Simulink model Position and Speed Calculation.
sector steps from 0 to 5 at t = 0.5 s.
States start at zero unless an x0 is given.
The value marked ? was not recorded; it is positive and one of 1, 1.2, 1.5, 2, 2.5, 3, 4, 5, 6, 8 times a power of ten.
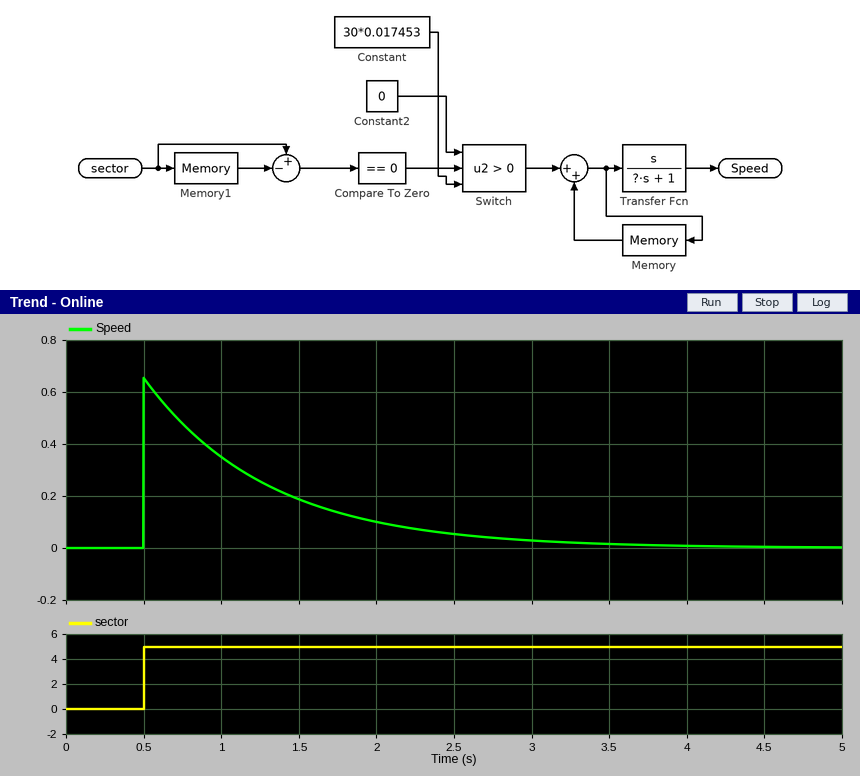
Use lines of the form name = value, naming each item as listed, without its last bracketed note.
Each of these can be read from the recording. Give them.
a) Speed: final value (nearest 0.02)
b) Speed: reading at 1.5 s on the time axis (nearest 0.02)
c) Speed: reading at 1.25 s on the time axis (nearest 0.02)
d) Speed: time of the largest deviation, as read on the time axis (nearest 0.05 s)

Speed: final value = 0.00
Speed: reading at 1.5 s on the time axis = 0.18
Speed: reading at 1.25 s on the time axis = 0.26
Speed: time of the largest deviation, as read on the time axis = 0.50 s
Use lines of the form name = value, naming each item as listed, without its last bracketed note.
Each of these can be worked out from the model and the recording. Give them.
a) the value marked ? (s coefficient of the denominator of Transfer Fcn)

the value marked ? = 0.8
